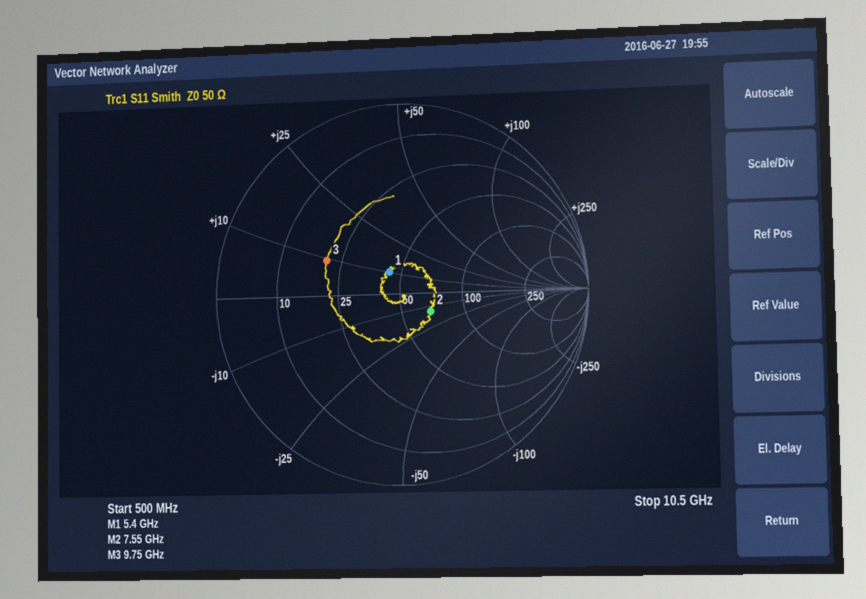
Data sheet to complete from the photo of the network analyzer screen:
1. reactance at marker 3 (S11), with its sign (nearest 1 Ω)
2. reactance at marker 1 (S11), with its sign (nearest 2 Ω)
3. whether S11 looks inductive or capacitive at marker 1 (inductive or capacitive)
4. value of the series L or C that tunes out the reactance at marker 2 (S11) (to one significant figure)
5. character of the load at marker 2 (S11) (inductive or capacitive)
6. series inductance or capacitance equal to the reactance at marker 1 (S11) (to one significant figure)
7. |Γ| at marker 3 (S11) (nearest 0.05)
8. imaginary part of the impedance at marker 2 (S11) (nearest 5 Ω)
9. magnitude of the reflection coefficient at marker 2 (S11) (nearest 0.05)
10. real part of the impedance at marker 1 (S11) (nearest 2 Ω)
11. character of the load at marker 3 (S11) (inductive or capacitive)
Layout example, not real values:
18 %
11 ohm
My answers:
+9 Ω
+10 Ω
inductive
300 pH
capacitive
300 pH
0.45
-15 Ω
0.20
44 Ω
inductive
